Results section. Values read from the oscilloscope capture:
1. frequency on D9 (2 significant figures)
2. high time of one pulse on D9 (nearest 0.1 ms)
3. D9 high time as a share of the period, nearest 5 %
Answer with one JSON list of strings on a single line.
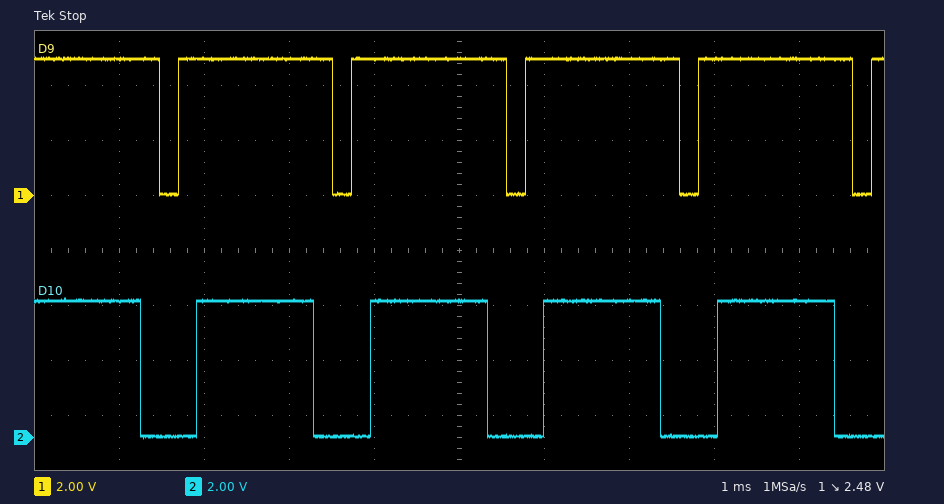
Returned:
["490 Hz", "1.8 ms", "90 %"]
